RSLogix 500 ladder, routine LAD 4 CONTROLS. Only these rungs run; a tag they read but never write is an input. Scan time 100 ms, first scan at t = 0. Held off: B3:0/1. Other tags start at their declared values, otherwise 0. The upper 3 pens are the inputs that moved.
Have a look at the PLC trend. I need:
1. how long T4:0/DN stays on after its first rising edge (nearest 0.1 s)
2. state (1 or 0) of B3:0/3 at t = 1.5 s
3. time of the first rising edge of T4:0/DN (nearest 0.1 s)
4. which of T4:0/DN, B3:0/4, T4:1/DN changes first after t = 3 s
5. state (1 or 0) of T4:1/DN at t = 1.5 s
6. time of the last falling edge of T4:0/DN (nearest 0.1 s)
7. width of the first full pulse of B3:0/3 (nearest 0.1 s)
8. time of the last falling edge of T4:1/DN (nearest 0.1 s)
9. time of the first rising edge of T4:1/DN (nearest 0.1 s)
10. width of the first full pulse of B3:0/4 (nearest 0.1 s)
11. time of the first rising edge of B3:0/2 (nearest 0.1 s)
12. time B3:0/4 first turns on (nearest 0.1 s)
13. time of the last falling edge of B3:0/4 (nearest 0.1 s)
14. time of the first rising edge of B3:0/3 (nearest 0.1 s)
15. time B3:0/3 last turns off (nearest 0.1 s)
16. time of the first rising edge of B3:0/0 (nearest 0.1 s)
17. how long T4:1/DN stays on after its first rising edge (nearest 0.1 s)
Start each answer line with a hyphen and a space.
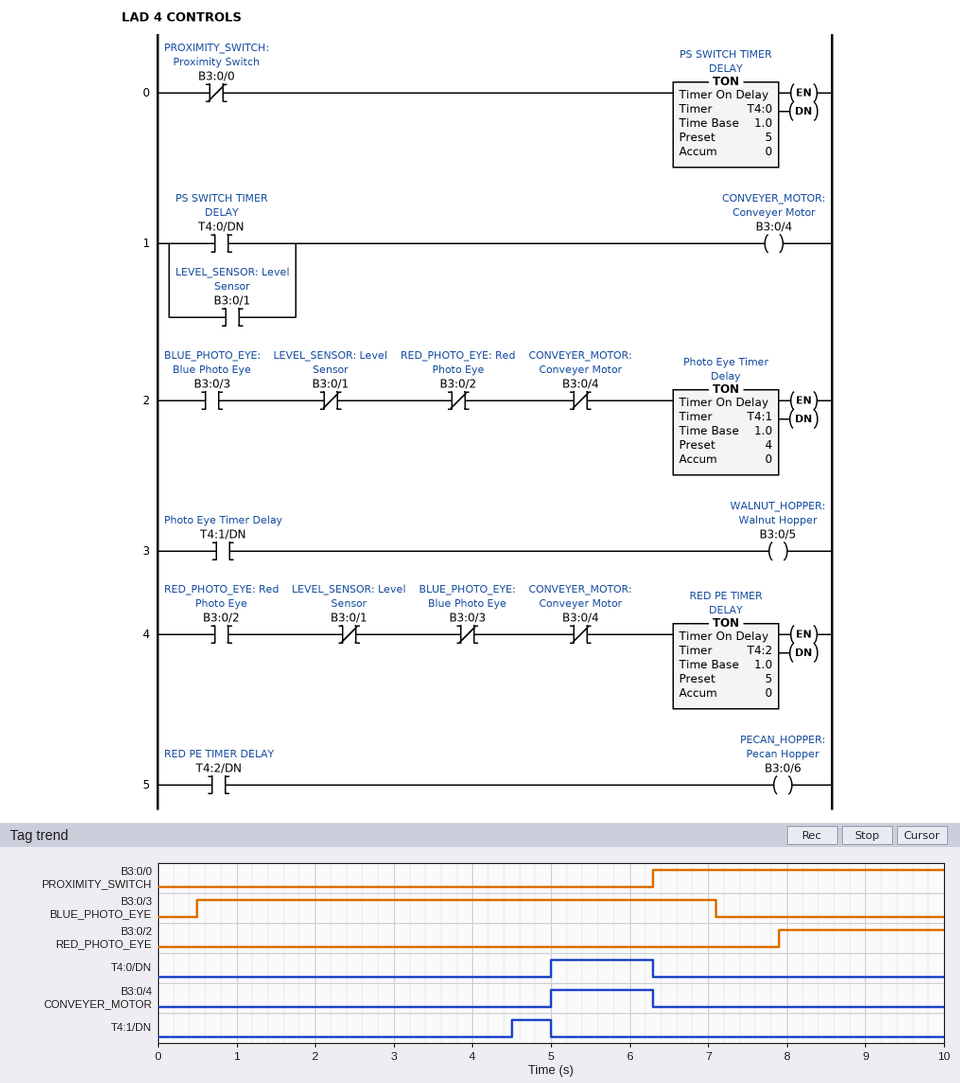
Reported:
- 1.3 s
- 1
- 5.0 s
- T4:1/DN
- 0
- 6.3 s
- 6.6 s
- 5.0 s
- 4.5 s
- 1.3 s
- 7.9 s
- 5.0 s
- 6.3 s
- 0.5 s
- 7.1 s
- 6.3 s
- 0.5 s
